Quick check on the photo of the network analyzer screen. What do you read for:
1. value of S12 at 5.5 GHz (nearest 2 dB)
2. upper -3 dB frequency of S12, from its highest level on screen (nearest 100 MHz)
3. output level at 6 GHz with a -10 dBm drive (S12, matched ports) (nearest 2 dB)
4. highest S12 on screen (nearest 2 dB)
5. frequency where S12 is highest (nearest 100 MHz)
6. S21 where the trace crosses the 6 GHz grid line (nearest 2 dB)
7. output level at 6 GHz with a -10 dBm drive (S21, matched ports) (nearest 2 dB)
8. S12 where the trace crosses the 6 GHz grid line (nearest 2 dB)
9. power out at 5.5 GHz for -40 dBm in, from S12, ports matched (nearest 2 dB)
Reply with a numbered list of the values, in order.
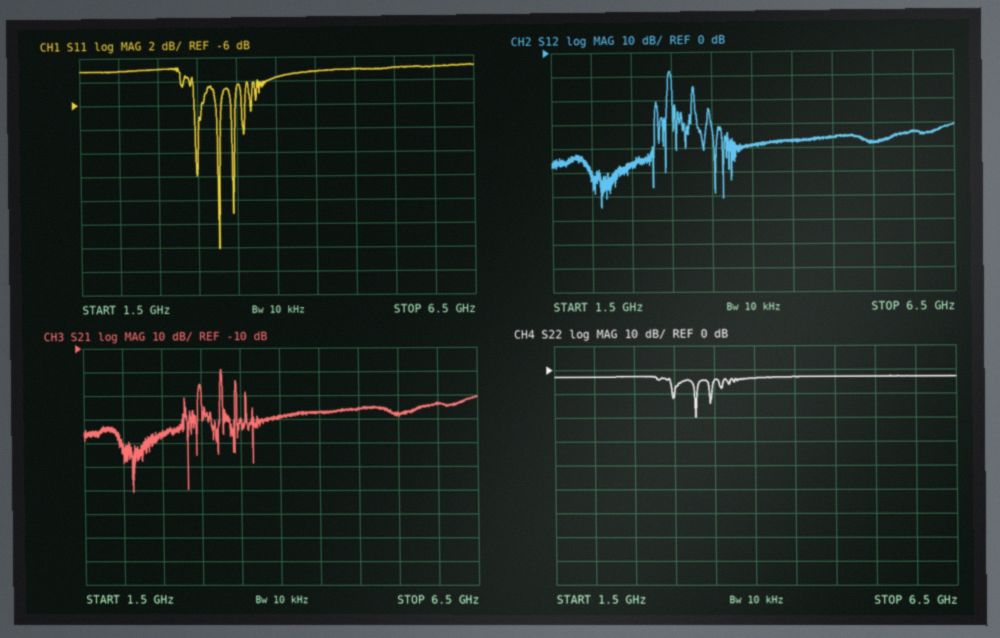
1. -38 dB
2. 3.0 GHz
3. -44 dBm
4. -8 dB
5. 3.0 GHz
6. -34 dB
7. -44 dBm
8. -34 dB
9. -78 dBm
